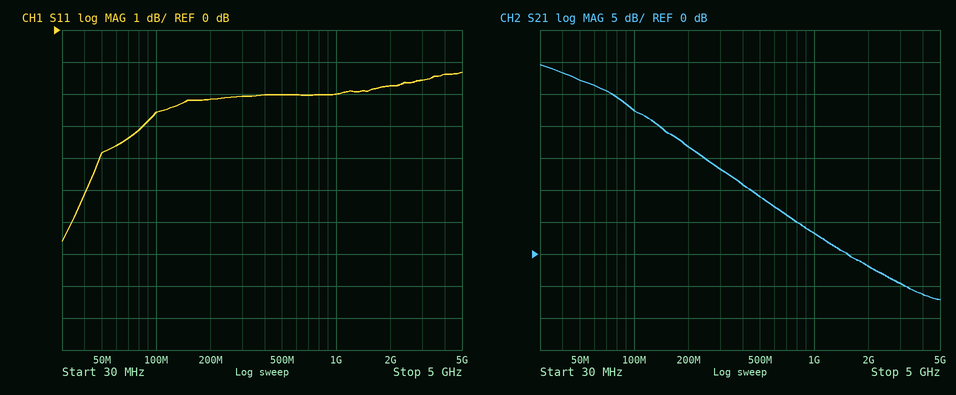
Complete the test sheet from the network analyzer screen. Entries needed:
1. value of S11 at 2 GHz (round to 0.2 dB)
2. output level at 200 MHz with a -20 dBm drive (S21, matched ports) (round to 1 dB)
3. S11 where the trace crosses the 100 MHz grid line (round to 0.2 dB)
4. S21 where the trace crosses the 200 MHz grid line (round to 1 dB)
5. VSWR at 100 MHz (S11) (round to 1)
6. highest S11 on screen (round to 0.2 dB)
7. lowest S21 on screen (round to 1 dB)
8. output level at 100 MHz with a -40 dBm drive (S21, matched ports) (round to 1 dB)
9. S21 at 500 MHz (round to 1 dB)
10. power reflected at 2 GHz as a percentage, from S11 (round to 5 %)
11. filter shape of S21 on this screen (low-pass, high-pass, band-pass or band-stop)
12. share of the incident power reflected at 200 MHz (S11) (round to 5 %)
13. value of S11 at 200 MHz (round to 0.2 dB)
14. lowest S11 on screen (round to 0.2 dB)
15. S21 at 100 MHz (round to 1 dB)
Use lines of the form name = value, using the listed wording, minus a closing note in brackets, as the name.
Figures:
value of S11 at 2 GHz = -1.8 dB
output level at 200 MHz with a -20 dBm drive (S21, matched ports) = -3 dBm
S11 where the trace crosses the 100 MHz grid line = -2.6 dB
S21 where the trace crosses the 200 MHz grid line = 17 dB
VSWR at 100 MHz (S11) = 7
highest S11 on screen = -1.4 dB
lowest S21 on screen = -7 dB
output level at 100 MHz with a -40 dBm drive (S21, matched ports) = -18 dBm
S21 at 500 MHz = 9 dB
power reflected at 2 GHz as a percentage, from S11 = 65 %
filter shape of S21 on this screen = low-pass
share of the incident power reflected at 200 MHz (S11) = 60 %
value of S11 at 200 MHz = -2.2 dB
lowest S11 on screen = -6.6 dB
S21 at 100 MHz = 22 dB
